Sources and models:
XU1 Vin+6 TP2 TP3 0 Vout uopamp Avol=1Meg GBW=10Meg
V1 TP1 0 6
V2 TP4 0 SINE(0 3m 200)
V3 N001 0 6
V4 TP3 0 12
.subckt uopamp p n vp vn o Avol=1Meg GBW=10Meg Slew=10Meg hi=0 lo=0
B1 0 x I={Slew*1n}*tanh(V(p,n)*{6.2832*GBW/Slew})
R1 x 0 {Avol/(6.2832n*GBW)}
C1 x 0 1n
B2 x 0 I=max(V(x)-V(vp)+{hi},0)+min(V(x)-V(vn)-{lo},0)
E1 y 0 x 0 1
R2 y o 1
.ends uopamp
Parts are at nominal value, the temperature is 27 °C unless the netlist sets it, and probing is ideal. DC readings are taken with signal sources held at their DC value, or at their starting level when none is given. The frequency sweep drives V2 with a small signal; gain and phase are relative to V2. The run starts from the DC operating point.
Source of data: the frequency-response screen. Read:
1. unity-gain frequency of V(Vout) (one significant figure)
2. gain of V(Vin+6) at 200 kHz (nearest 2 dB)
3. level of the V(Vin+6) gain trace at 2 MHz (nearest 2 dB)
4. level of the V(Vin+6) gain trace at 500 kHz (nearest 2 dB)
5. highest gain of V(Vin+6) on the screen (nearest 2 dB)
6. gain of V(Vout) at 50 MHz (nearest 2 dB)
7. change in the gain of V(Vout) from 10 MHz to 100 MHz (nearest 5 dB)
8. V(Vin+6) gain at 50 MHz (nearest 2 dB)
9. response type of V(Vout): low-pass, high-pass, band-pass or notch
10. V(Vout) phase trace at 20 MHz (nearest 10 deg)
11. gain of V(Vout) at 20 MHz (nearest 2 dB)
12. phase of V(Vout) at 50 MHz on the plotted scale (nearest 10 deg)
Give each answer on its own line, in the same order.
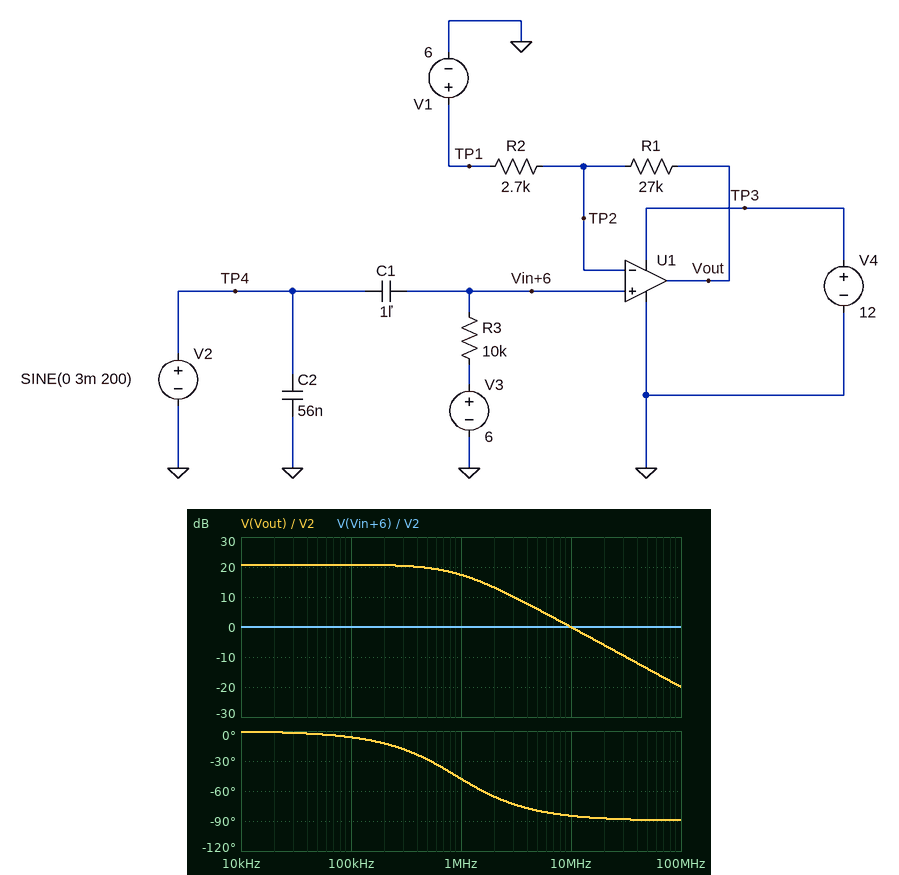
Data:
10 MHz
0 dB
0 dB
0 dB
0 dB
-14 dB
-20 dB
0 dB
low-pass
-90 deg
-6 dB
-90 deg
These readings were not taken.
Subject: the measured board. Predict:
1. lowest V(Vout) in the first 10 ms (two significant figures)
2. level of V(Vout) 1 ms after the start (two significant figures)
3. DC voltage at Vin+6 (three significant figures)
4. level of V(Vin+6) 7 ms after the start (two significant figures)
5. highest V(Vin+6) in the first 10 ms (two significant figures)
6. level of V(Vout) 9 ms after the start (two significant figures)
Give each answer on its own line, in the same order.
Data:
6.0 V
6.0 V
6.00 V
6.0 V
6.0 V
6.0 V
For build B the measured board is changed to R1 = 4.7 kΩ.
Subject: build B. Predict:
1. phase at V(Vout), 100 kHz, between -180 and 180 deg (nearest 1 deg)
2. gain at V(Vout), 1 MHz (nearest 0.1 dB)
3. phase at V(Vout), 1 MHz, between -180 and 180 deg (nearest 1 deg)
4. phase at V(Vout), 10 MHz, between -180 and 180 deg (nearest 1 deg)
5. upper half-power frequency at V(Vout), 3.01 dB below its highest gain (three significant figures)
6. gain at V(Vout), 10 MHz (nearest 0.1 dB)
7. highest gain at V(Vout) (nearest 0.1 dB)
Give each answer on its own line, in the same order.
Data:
-2 deg
8.4 dB
-15 deg
-70 deg
3.65 MHz
-0.5 dB
8.8 dB
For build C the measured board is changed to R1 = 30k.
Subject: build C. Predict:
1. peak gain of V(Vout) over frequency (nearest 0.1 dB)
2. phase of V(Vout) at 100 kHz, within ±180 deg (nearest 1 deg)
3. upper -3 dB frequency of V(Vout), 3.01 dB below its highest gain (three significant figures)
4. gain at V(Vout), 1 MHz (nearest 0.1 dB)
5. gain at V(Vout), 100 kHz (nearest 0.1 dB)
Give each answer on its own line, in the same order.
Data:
21.7 dB
-7 deg
826 kHz
17.7 dB
21.6 dB
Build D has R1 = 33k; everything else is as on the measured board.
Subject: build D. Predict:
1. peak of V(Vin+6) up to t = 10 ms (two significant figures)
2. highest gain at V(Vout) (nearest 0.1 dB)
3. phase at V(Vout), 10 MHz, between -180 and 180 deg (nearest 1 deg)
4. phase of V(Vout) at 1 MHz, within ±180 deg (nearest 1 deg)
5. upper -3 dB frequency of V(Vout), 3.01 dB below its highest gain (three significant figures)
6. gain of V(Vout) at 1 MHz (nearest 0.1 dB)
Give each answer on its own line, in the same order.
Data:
6.0 V
22.4 dB
-86 deg
-53 deg
756 kHz
18.0 dB
